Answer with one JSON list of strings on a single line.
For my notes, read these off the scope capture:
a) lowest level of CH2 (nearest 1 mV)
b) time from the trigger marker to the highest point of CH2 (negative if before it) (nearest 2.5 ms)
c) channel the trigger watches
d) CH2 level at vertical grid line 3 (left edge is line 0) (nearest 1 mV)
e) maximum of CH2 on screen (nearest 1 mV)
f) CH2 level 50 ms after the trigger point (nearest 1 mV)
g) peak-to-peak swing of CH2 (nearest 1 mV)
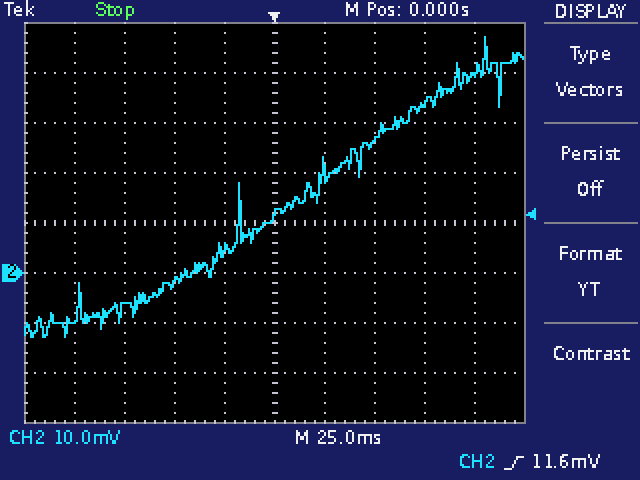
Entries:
["-13 mV", "+105.0 ms", "CH2", "-2 mV", "47 mV", "26 mV", "60 mV"]
